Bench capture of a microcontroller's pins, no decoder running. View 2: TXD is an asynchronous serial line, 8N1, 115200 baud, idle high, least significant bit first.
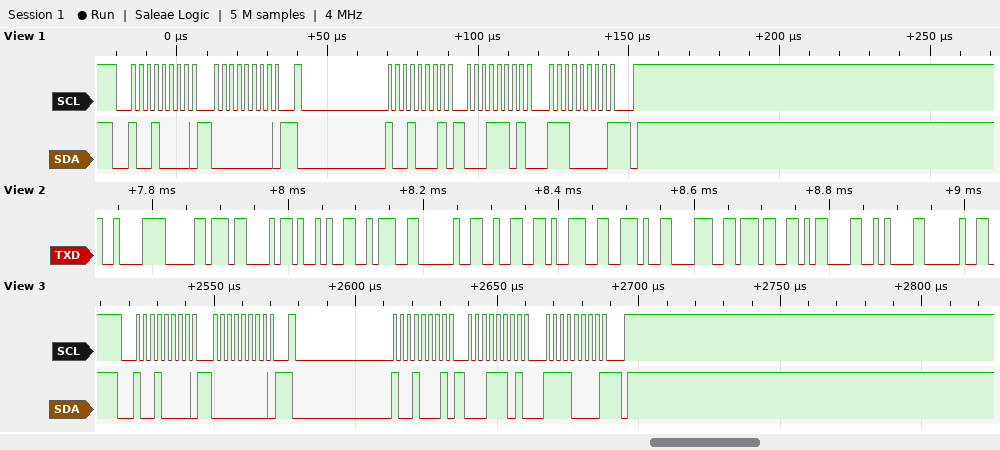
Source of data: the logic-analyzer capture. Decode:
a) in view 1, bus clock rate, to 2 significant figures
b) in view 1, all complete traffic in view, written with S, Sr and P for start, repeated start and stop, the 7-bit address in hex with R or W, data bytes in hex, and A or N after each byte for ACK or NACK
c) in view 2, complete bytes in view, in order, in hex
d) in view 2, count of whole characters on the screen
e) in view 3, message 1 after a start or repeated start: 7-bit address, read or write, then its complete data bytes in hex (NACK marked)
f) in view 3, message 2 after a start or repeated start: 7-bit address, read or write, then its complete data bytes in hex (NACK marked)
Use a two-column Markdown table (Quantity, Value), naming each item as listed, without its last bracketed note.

| Quantity | Value |
|---|---|
| in view 1, bus clock rate, to 2 significant figures | 400 kHz |
| in view 1, all complete traffic in view, written with S, Sr and P for start, repeated start and stop, the 7-bit address in hex with R or W, data bytes in hex, and A or N after each byte for ACK or NACK | S 48W A 00 A Sr 48R A 1D A E0 N P |
| in view 2, complete bytes in view, in order, in hex | 0xC2 0xB0 0x43 0x29 0x3A 0x20 0x32 0x39 0x2E 0x38 0x37 0x0D 0x0A 0x20 |
| in view 2, count of whole characters on the screen | 14 |
| in view 3, message 1 after a start or repeated start: 7-bit address, read or write, then its complete data bytes in hex | 0x48 write: 00 |
| in view 3, message 2 after a start or repeated start: 7-bit address, read or write, then its complete data bytes in hex | 0x48 read: 1D F0 NACK |
